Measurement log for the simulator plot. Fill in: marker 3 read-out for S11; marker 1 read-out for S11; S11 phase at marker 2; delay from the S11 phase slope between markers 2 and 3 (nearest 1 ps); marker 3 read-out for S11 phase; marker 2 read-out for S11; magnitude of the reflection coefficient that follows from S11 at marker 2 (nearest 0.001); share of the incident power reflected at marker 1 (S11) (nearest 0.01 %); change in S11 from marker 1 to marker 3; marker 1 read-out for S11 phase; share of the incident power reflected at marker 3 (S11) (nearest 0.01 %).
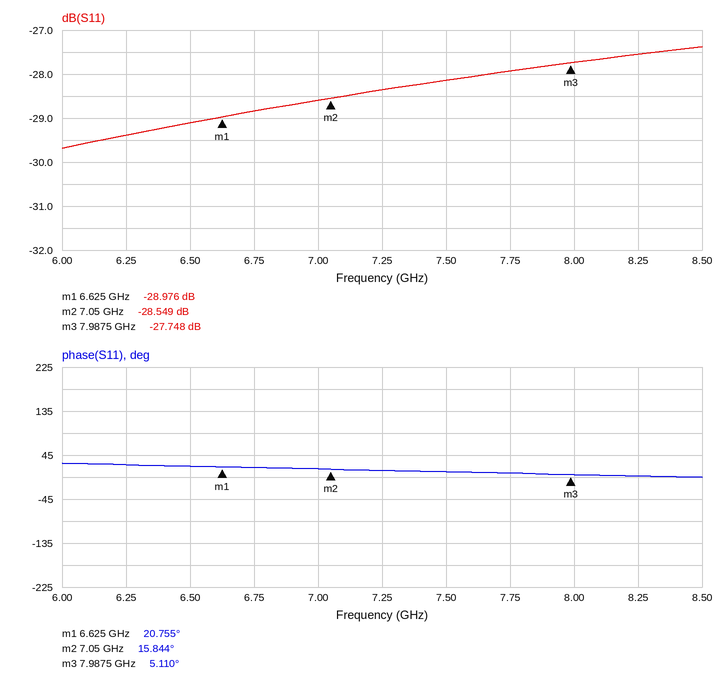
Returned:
-27.748 dB
-28.976 dB
15.844°
32 ps
5.110°
-28.549 dB
0.037
0.13 %
1.228 dB
20.755°
0.17 %
